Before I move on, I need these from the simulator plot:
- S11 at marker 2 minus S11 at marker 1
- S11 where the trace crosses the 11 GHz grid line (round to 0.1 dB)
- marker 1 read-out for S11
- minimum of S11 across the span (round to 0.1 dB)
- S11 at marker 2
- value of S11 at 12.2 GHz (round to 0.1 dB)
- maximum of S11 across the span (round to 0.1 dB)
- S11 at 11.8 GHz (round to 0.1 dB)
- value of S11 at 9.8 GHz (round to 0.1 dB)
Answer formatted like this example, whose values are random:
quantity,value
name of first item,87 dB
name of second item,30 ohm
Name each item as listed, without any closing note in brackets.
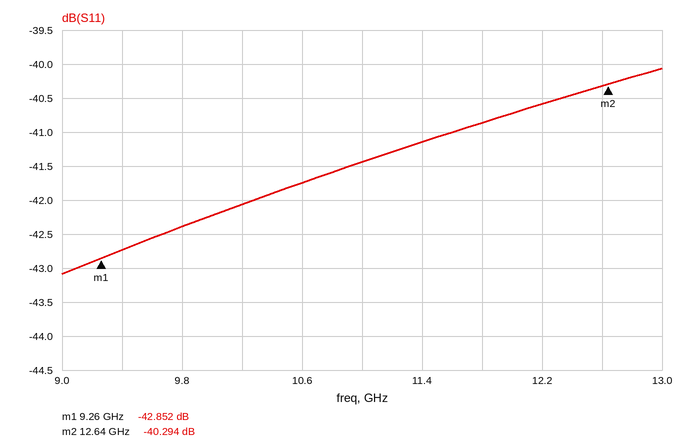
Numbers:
quantity,value
S11 at marker 2 minus S11 at marker 1,2.558 dB
S11 where the trace crosses the 11 GHz grid line,-41.4 dB
marker 1 read-out for S11,-42.852 dB
minimum of S11 across the span,-43.1 dB
S11 at marker 2,-40.294 dB
value of S11 at 12.2 GHz,-40.6 dB
maximum of S11 across the span,-40.1 dB
S11 at 11.8 GHz,-40.9 dB
value of S11 at 9.8 GHz,-42.4 dB
